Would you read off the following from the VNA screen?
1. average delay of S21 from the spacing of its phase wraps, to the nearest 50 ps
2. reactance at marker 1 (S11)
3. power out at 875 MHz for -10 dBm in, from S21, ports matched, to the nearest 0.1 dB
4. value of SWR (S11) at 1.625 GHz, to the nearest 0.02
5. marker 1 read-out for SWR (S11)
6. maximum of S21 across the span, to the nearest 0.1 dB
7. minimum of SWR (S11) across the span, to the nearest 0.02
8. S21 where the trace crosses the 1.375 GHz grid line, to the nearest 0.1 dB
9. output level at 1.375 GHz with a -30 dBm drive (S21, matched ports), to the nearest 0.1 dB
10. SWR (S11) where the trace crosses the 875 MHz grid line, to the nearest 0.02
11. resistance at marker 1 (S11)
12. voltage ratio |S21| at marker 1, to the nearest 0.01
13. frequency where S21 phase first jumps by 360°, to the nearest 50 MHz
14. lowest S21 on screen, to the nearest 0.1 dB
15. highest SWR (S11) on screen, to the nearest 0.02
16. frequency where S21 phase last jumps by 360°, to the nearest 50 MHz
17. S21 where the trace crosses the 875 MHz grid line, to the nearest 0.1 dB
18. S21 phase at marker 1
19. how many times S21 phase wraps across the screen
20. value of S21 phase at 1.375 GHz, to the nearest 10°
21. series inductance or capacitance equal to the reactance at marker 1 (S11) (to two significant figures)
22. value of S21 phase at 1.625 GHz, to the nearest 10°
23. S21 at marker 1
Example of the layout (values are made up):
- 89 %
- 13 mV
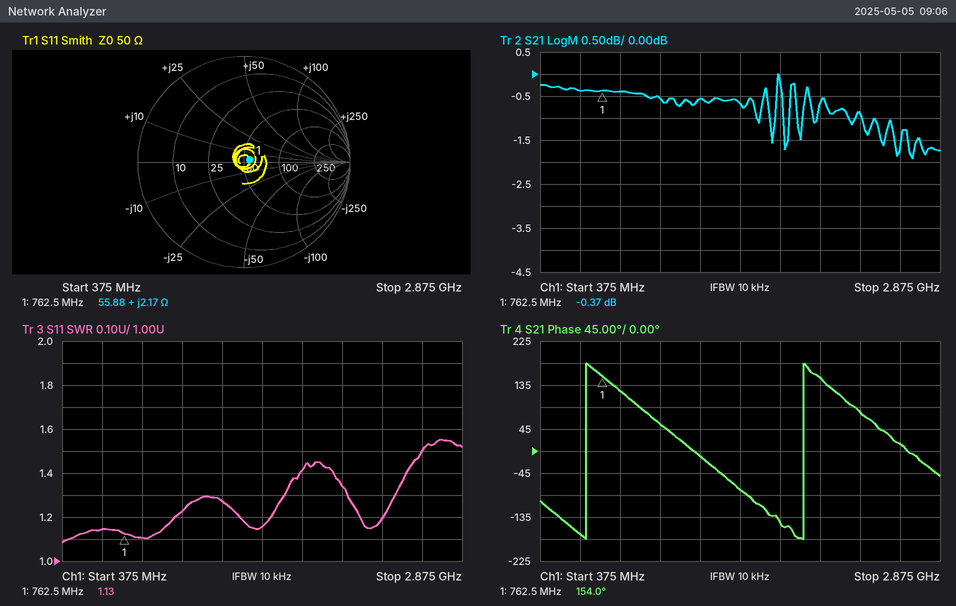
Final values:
- 750 ps
- +2.17 Ω
- -10.4 dBm
- 1.16
- 1.13
- 0.0 dB
- 1.08
- -0.6 dB
- -30.6 dBm
- 1.10
- 55.88 Ω
- 0.96
- 650 MHz
- -1.9 dB
- 1.56
- 2.00 GHz
- -0.4 dB
- 154.0°
- 2
- -10°
- 450 pH
- -80°
- -0.37 dB
